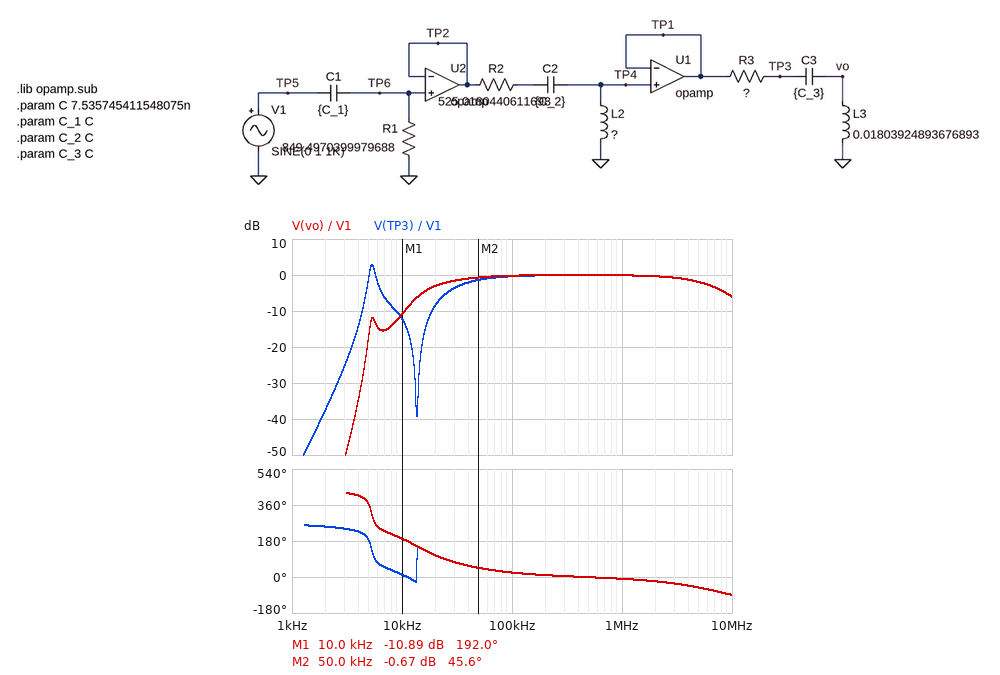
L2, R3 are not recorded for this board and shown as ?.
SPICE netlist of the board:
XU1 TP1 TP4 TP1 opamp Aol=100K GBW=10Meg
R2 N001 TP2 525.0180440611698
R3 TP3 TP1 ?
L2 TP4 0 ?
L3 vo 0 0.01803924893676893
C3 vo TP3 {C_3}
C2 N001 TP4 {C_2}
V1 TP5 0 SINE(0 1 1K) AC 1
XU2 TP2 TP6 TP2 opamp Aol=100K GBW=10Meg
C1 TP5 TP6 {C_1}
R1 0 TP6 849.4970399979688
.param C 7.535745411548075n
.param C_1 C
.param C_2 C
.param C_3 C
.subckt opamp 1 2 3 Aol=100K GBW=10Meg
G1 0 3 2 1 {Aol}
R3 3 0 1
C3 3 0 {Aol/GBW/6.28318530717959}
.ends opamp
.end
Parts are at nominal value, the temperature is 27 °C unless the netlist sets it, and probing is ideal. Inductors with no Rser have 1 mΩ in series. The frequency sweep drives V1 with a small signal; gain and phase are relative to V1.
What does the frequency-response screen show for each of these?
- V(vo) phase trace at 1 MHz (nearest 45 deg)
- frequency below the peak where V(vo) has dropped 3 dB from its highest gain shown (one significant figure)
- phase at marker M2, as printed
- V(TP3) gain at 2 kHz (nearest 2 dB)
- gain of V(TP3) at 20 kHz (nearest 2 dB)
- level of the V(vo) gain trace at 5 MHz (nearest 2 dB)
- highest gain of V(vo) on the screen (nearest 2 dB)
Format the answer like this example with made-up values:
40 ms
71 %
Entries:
0 deg
20 kHz
45.6 deg
-38 dB
-8 dB
-2 dB
0 dB
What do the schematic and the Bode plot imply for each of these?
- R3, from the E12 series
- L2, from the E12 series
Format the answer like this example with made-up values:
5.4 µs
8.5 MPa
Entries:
1.8 kΩ
120 mH
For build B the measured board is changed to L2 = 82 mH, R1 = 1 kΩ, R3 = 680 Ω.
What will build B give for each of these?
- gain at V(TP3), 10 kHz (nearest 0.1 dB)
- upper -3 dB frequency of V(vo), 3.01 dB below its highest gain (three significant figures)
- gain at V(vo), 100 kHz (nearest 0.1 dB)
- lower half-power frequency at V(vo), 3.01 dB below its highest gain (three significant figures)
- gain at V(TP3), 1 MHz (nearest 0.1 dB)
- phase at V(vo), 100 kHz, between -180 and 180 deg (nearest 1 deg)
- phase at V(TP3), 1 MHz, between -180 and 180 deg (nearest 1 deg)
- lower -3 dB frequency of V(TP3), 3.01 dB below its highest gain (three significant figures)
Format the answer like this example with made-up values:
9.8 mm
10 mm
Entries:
-4.6 dB
22.5 kHz
0 dB
11.9 kHz
-0.1 dB
15 deg
-10 deg
6.03 kHz
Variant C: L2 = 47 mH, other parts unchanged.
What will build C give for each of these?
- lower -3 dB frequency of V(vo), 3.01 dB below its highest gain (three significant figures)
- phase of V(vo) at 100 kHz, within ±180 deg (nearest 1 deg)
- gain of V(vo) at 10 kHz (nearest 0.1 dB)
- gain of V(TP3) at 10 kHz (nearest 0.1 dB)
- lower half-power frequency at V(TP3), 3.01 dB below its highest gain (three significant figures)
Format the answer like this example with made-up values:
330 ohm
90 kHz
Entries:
15.4 kHz
23 deg
-4.2 dB
-5.5 dB
7.73 kHz
